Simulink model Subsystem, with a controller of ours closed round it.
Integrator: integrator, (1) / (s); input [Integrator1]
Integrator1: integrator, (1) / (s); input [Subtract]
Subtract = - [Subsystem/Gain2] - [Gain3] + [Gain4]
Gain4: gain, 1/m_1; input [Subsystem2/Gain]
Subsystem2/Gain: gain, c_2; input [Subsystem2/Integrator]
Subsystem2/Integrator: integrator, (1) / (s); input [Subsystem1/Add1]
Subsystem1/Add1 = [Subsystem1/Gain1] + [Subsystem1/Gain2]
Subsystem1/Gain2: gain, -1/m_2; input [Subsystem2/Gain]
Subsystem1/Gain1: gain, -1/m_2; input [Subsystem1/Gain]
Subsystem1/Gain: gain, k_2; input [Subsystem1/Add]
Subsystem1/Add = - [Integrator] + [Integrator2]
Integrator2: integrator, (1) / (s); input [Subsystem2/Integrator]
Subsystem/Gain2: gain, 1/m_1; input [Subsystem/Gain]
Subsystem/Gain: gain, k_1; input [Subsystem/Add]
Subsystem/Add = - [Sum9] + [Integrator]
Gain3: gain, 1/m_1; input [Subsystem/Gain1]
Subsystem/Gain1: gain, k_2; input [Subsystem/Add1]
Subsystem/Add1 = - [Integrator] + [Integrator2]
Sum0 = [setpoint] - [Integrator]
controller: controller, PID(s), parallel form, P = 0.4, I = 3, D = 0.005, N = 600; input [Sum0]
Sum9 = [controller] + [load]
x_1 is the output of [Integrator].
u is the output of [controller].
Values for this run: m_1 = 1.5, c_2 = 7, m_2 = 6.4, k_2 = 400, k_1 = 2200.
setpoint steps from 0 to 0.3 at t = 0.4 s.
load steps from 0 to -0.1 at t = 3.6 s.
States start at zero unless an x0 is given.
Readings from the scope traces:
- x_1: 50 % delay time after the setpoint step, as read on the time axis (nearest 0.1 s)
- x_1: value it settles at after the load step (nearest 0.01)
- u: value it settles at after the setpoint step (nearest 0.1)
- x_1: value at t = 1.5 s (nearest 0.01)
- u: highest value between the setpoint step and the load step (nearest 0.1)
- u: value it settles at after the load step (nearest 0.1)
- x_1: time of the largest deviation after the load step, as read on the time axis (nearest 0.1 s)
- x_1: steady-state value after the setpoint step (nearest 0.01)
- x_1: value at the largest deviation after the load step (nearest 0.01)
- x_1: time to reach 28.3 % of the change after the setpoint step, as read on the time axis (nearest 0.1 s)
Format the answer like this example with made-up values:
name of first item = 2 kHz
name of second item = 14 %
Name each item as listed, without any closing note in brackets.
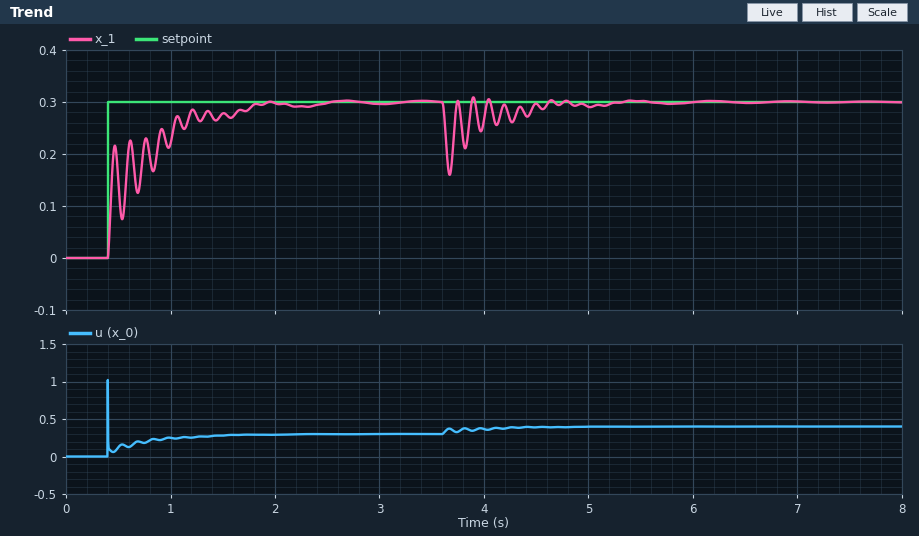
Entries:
x_1: 50 % delay time after the setpoint step, as read on the time axis = 0.4 s
x_1: value it settles at after the load step = 0.30
u: value it settles at after the setpoint step = 0.3
x_1: value at t = 1.5 s = 0.28
u: highest value between the setpoint step and the load step = 1.0
u: value it settles at after the load step = 0.4
x_1: time of the largest deviation after the load step, as read on the time axis = 3.7 s
x_1: steady-state value after the setpoint step = 0.30
x_1: value at the largest deviation after the load step = 0.16
x_1: time to reach 28.3 % of the change after the setpoint step, as read on the time axis = 0.4 s
